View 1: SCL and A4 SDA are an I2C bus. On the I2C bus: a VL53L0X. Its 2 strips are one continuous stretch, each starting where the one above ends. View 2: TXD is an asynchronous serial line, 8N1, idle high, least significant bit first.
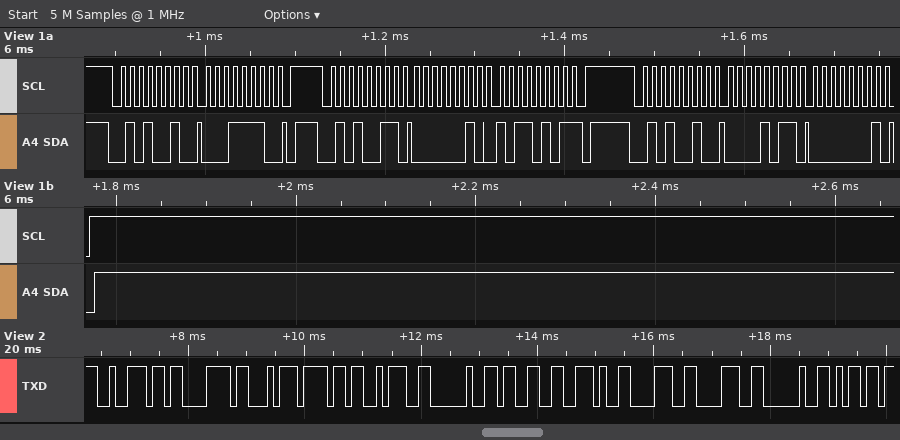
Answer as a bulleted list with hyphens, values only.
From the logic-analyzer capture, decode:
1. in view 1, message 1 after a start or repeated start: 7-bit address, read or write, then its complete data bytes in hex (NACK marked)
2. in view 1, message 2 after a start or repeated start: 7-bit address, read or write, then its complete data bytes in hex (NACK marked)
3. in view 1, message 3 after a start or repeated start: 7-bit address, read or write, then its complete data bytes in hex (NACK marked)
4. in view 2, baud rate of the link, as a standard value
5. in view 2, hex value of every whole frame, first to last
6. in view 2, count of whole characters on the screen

- 0x29 write: 1E
- 0x29 read: 02 B5 NACK
- 0x29 write: 0B 01
- 9600 baud
- 72 C3 A3 6F 3A 20 33 2E 38 38 20 6D
- 12
